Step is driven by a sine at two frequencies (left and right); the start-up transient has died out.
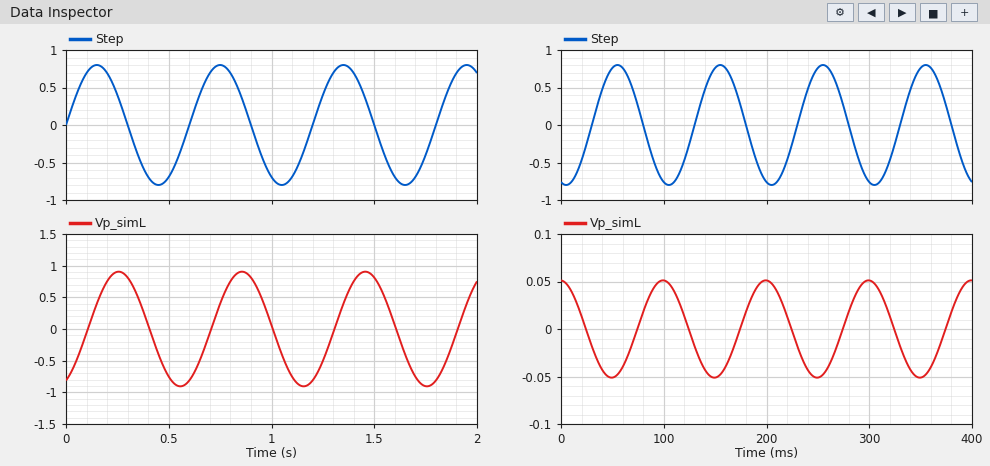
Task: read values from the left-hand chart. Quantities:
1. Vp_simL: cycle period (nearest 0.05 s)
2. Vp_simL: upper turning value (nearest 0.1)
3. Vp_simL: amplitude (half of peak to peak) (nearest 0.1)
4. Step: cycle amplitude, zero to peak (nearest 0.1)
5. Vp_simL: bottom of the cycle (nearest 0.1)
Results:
0.60 s
0.9
0.9
0.8
-0.9
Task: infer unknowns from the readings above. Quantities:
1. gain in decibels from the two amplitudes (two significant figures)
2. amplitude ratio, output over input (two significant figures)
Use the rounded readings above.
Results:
1.0 dB
1.1
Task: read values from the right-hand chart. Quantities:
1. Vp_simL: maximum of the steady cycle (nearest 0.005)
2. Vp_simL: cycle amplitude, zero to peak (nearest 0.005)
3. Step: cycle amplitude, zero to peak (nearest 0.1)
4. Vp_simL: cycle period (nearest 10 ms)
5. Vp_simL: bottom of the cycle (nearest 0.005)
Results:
0.050
0.050
0.8
100 ms
-0.050
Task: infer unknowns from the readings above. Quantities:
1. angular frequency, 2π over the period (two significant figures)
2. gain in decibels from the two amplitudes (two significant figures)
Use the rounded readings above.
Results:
0.063 rad/ms
-24 dB
